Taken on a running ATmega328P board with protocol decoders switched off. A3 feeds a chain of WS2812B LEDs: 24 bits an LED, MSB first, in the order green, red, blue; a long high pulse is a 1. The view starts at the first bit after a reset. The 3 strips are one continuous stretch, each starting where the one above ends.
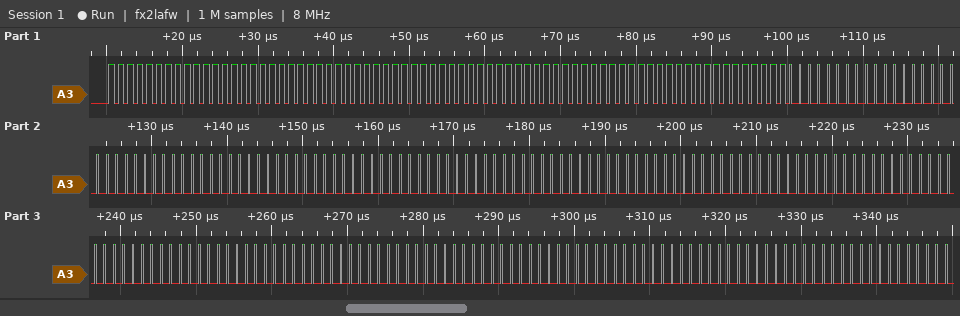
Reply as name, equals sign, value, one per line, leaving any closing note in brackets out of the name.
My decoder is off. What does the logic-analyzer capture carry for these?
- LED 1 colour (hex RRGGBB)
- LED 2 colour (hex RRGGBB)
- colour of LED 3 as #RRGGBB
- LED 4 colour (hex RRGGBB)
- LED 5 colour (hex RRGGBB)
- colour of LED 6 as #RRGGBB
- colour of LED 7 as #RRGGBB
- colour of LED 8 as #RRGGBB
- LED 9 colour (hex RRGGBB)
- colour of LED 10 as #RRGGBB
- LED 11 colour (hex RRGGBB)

LED 1 colour = #FFFFFF
LED 2 colour = #FFFFFF
colour of LED 3 as #RRGGBB = #FFFFFF
LED 4 colour = #000000
LED 5 colour = #000000
colour of LED 6 as #RRGGBB = #000000
colour of LED 7 as #RRGGBB = #000000
colour of LED 8 as #RRGGBB = #000000
LED 9 colour = #000000
colour of LED 10 as #RRGGBB = #000000
LED 11 colour = #000000
